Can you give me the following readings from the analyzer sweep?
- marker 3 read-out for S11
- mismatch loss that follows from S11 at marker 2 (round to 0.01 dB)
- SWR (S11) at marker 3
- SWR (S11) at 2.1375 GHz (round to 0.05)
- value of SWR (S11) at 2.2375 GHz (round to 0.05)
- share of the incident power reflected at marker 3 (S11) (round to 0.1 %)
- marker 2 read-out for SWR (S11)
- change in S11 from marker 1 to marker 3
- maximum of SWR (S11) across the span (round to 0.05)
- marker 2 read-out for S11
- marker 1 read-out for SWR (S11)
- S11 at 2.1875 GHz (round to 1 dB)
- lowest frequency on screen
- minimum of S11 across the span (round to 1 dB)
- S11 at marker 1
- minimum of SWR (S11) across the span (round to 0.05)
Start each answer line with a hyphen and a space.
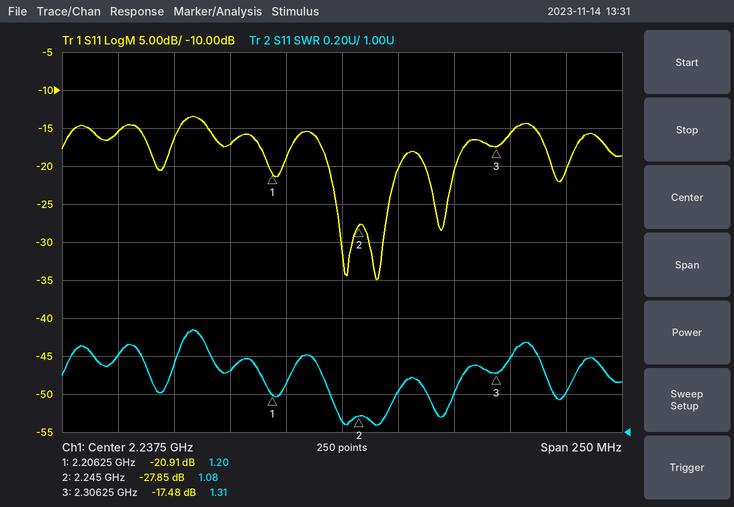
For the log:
- -17.48 dB
- 0.01 dB
- 1.31
- 1.40
- 1.05
- 1.8 %
- 1.08
- 3.43 dB
- 1.55
- -27.85 dB
- 1.20
- -17 dB
- 2.1125 GHz
- -35 dB
- -20.91 dB
- 1.05
